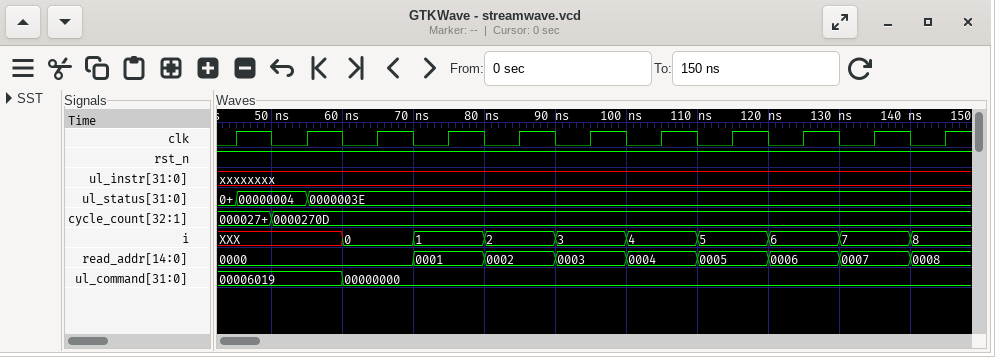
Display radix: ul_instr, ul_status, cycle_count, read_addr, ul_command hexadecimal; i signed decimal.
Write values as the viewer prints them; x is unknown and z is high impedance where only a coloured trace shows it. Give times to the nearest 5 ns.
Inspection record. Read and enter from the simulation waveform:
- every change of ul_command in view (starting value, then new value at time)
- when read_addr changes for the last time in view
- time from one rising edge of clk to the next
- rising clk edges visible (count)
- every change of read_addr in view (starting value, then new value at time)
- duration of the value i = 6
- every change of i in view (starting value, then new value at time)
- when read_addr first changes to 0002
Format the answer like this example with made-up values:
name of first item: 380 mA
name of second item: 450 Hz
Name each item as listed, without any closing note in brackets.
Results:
every change of ul_command in view: 00006019, 00000000 at 60 ns
when read_addr changes for the last time in view: 140 ns
time from one rising edge of clk to the next: 10 ns
rising clk edges visible: 11
every change of read_addr in view: 0000, 0001 at 70 ns, 0002 at 80 ns, 0003 at 90 ns, 0004 at 100 ns, 0005 at 110 ns, 0006 at 120 ns, 0007 at 130 ns, 0008 at 140 ns
duration of the value i = 6: 10 ns
every change of i in view: XXX, 0 at 60 ns, 1 at 70 ns, 2 at 80 ns, 3 at 90 ns, 4 at 100 ns, 5 at 110 ns, 6 at 120 ns, 7 at 130 ns, 8 at 140 ns
when read_addr first changes to 0002: 80 ns
